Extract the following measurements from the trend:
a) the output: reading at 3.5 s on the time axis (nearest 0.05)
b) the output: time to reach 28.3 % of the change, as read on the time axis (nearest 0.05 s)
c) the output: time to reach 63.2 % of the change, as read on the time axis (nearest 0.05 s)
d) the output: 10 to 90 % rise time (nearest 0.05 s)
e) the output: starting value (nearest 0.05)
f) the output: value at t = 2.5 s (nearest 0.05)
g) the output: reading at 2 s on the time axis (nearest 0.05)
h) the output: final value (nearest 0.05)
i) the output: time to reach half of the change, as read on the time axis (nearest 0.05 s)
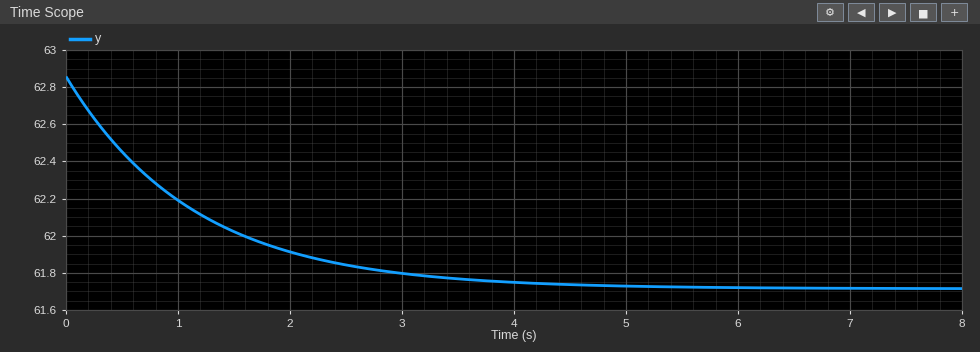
61.75
0.40 s
1.15 s
2.50 s
62.85
61.85
61.90
61.70
0.80 s
